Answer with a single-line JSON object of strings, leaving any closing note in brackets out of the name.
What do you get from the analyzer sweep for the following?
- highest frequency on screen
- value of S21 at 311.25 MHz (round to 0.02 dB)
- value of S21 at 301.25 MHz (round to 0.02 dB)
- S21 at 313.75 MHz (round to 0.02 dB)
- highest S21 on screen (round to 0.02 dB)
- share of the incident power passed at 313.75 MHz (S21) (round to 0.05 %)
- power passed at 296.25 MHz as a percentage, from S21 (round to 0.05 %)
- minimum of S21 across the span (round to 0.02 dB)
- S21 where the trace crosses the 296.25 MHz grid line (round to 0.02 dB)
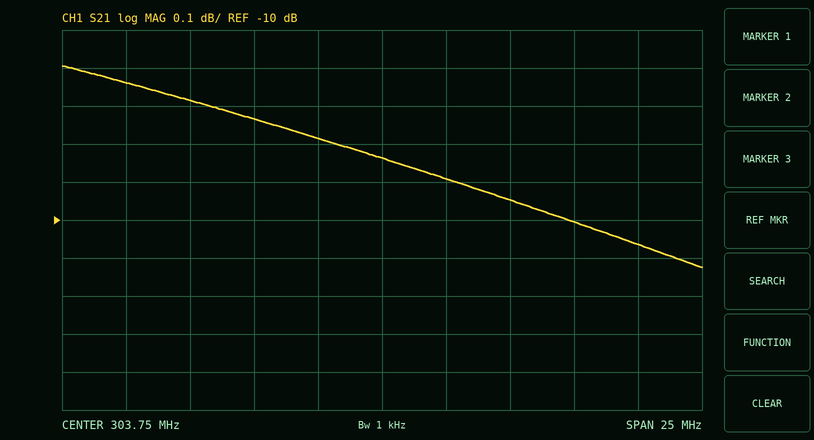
{"highest frequency on screen": "316.25 MHz", "value of S21 at 311.25 MHz": "-10.00 dB", "value of S21 at 301.25 MHz": "-9.78 dB", "S21 at 313.75 MHz": "-10.06 dB", "highest S21 on screen": "-9.60 dB", "share of the incident power passed at 313.75 MHz (S21)": "9.85 %", "power passed at 296.25 MHz as a percentage, from S21": "10.75 %", "minimum of S21 across the span": "-10.12 dB", "S21 where the trace crosses the 296.25 MHz grid line": "-9.68 dB"}
